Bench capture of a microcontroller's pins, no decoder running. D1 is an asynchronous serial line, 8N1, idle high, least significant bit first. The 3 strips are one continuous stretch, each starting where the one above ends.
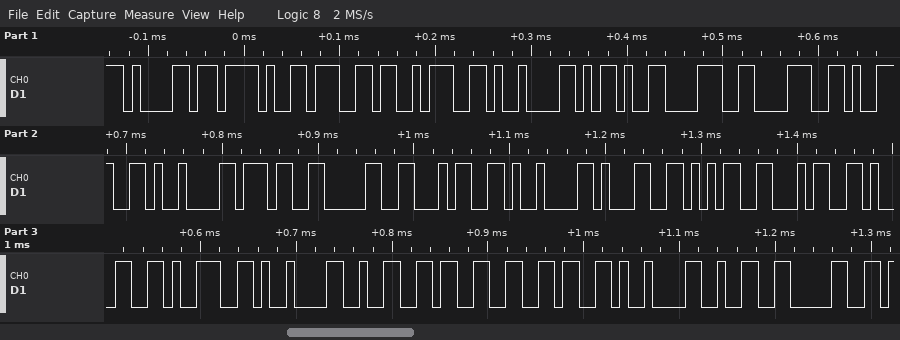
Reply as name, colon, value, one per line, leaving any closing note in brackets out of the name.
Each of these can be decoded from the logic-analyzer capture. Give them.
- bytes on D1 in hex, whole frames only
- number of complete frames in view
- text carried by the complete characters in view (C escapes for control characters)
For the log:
bytes on D1 in hex, whole frames only: 0x61 0x2F 0x67 0x3A 0x09 0x2D 0x38 0x38 0x39 0x09 0x37 0x30 0x34 0x09 0x31 0x35 0x34 0x31 0x39 0x09 0x32 0x33 0x36 0x09 0x32 0x30
number of complete frames in view: 26
text carried by the complete characters in view: "a/g:\t-889\t704\t15419\t236\t20"
